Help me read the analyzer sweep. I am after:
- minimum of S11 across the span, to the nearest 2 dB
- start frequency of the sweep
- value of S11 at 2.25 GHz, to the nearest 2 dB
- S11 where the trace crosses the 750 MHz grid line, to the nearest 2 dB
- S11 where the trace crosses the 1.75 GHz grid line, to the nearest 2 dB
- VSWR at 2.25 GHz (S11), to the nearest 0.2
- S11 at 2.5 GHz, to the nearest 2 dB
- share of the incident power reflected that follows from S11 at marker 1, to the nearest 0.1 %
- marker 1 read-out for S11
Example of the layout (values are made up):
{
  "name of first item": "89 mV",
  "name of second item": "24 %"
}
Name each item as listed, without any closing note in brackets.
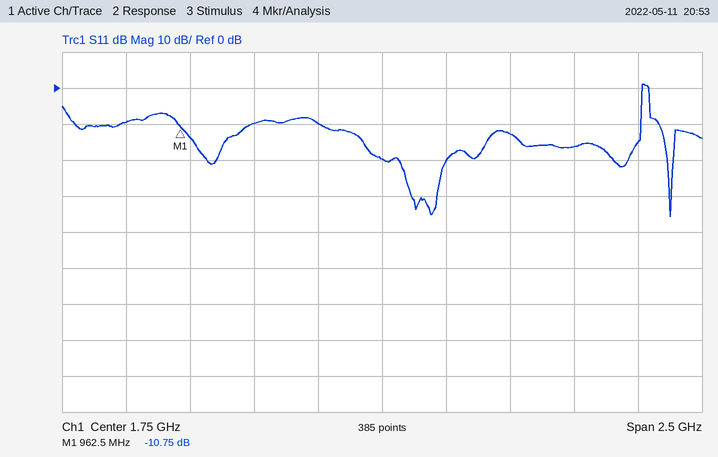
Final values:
{
  "minimum of S11 across the span, to the nearest 2 dB": "-36 dB",
  "start frequency of the sweep": "500 MHz",
  "value of S11 at 2.25 GHz, to the nearest 2 dB": "-12 dB",
  "S11 where the trace crosses the 750 MHz grid line, to the nearest 2 dB": "-10 dB",
  "S11 where the trace crosses the 1.75 GHz grid line, to the nearest 2 dB": "-20 dB",
  "VSWR at 2.25 GHz (S11), to the nearest 0.2": "1.6",
  "S11 at 2.5 GHz, to the nearest 2 dB": "-16 dB",
  "share of the incident power reflected that follows from S11 at marker 1, to the nearest 0.1 %": "8.4 %",
  "marker 1 read-out for S11": "-10.75 dB"
}
